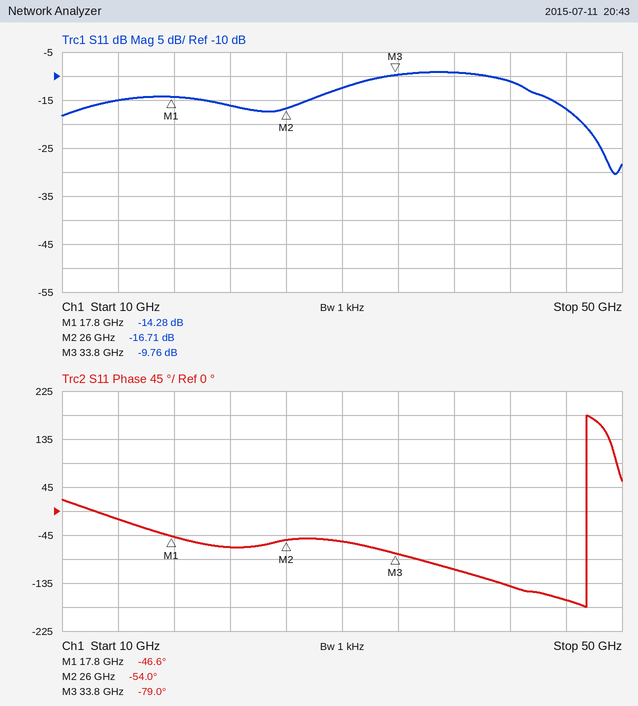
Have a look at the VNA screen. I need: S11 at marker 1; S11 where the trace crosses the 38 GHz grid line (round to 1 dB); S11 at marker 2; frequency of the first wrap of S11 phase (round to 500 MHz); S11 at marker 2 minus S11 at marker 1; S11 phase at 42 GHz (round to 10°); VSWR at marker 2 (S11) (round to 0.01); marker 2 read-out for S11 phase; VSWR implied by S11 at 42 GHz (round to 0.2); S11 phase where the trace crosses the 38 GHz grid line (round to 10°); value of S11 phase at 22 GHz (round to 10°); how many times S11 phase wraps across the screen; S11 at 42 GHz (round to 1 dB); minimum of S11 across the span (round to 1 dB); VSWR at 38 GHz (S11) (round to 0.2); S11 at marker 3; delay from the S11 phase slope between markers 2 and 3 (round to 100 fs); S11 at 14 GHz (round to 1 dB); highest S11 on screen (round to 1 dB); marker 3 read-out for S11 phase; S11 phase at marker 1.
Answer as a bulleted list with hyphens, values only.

- -14.28 dB
- -9 dB
- -16.71 dB
- 47.5 GHz
- -2.43 dB
- -140°
- 1.34
- -54.0°
- 1.8
- -110°
- -70°
- 1
- -11 dB
- -30 dB
- 2.0
- -9.76 dB
- 8.9 ps
- -15 dB
- -9 dB
- -79.0°
- -46.6°
